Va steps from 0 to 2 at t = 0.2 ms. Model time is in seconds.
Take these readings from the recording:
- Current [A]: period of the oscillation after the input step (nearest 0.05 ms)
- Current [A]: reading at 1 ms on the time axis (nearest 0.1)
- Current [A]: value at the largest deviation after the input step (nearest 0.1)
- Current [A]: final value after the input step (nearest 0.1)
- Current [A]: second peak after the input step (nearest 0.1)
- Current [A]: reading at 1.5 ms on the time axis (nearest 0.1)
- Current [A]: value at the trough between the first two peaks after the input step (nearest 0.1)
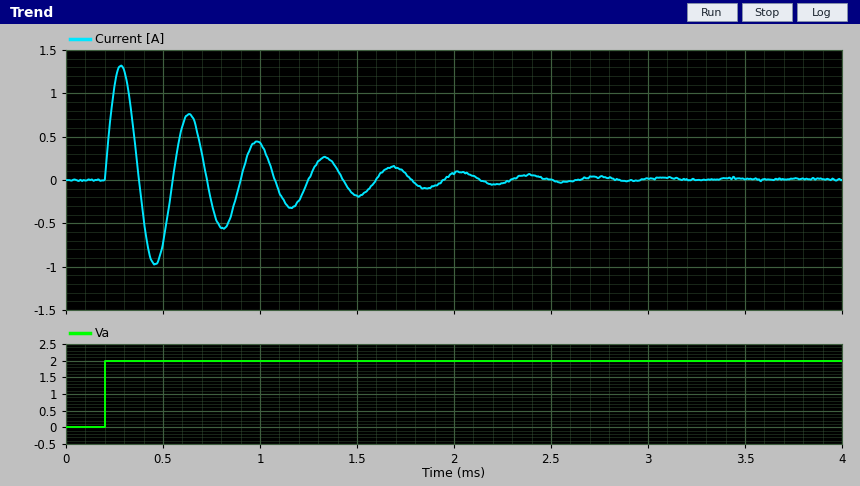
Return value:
0.35 ms
0.4
1.3
0.0
0.8
-0.2
-1.0
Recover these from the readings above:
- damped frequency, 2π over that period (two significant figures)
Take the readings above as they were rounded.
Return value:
18 rad/ms
